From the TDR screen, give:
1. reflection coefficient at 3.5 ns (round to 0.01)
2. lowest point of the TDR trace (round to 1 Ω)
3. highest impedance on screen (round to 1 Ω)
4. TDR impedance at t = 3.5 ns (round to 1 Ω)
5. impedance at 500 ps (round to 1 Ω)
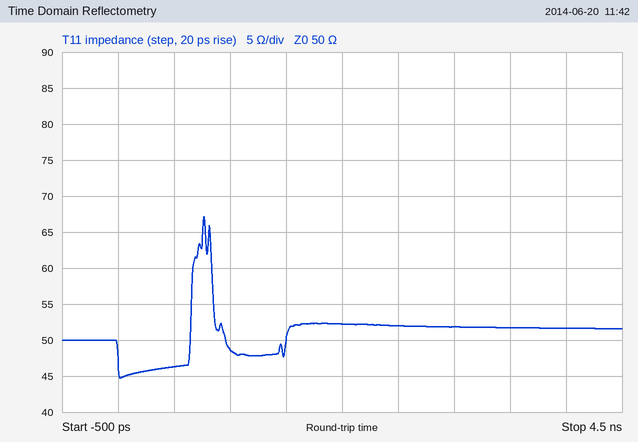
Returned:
+0.02
45 Ω
67 Ω
52 Ω
46 Ω
